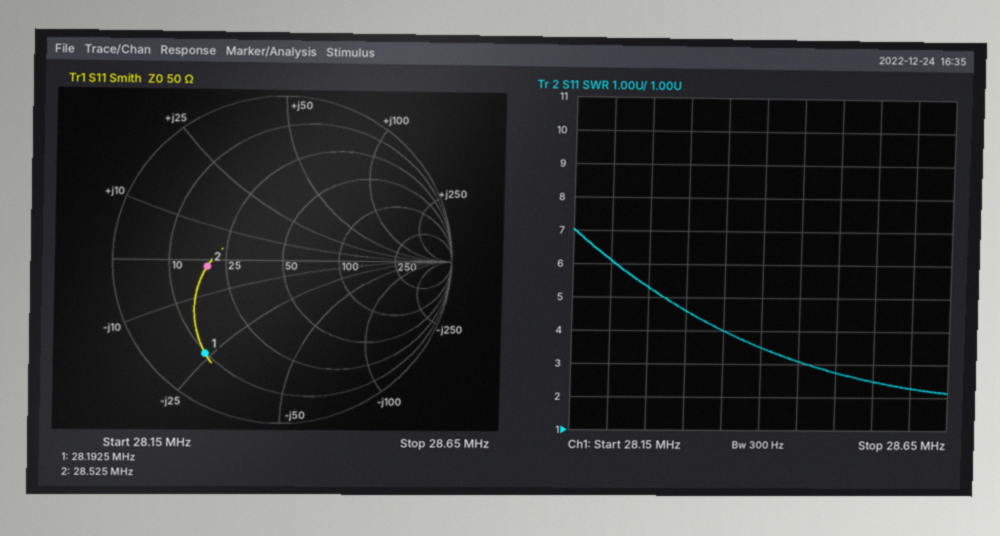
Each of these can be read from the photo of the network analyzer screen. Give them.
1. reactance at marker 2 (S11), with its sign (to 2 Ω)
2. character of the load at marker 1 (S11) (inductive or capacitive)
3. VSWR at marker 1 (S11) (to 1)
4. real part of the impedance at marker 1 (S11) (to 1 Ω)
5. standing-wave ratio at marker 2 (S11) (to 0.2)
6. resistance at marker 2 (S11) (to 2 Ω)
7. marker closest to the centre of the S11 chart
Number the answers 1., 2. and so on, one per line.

1. -2 Ω
2. capacitive
3. 6
4. 10 Ω
5. 2.6
6. 20 Ω
7. marker 2
